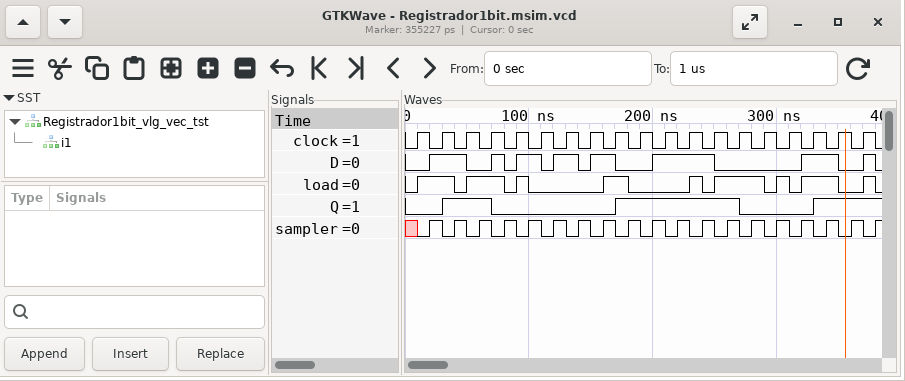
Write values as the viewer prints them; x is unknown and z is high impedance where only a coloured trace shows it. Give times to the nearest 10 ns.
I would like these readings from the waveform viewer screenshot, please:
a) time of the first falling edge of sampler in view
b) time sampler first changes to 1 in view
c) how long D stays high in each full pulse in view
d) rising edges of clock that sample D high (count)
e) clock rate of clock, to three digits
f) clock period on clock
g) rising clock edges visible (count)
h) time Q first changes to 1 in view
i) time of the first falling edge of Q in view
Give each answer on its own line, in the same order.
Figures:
30 ns
20 ns
30 ns, 10 ns, 20 ns, 20 ns, 20 ns, 50 ns, 30 ns, 10 ns
10
50.0 MHz
20 ns
19
30 ns
70 ns
